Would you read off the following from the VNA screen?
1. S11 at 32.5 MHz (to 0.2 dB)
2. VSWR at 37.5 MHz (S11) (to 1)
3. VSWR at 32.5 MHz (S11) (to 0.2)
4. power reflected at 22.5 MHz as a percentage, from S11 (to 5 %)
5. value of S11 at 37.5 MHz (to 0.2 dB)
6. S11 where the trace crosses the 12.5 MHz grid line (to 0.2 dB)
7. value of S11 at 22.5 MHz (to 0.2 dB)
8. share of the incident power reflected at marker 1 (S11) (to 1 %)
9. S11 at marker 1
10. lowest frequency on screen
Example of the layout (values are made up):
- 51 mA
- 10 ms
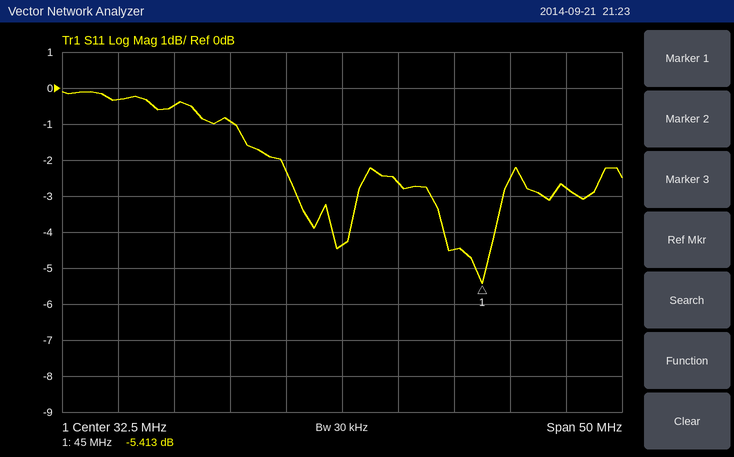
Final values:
- -4.4 dB
- 7
- 4.0
- 80 %
- -2.6 dB
- -0.4 dB
- -1.0 dB
- 29 %
- -5.413 dB
- 7.5 MHz
